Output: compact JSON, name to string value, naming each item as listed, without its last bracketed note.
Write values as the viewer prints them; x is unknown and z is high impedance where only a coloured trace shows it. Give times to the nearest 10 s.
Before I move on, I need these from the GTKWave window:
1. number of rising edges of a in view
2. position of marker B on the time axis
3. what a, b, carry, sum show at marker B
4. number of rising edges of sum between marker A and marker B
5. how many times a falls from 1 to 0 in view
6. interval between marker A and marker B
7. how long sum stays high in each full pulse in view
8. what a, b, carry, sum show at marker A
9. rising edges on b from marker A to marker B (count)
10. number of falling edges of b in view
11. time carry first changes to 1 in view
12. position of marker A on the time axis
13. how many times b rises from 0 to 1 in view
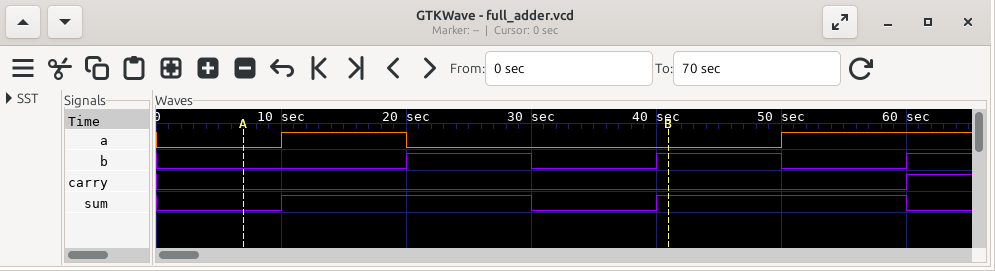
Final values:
{"number of rising edges of a in view": "2", "position of marker B on the time axis": "40 s", "what a, b, carry, sum show at marker B": "a=0, b=1, carry=0, sum=1", "number of rising edges of sum between marker A and marker B": "2", "how many times a falls from 1 to 0 in view": "1", "interval between marker A and marker B": "30 s", "how long sum stays high in each full pulse in view": "20 s, 20 s", "what a, b, carry, sum show at marker A": "a=0, b=0, carry=0, sum=0", "rising edges on b from marker A to marker B": "2", "number of falling edges of b in view": "2", "time carry first changes to 1 in view": "60 s", "position of marker A on the time axis": "10 s", "how many times b rises from 0 to 1 in view": "3"}
